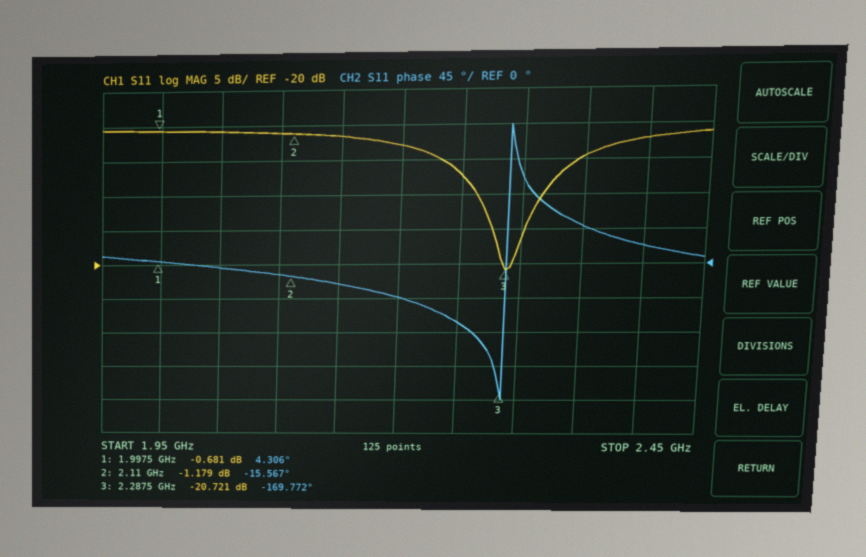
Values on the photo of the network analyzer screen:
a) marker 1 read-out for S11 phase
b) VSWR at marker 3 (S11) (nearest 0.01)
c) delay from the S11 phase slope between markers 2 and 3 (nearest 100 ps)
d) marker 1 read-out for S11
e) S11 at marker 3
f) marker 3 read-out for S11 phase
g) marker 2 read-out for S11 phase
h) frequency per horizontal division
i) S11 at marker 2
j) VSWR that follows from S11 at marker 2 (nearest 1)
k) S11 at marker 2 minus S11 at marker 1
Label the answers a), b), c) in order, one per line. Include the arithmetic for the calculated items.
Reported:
a) 4.306°
b) (1 + 0.0920)/(1 − 0.0920) ≈ 1.20
c) −(-169.772° − (-15.567°))/(360° × 177.5 MHz) ≈ 2.4 ns
d) -0.681 dB
e) -20.721 dB
f) -169.772°
g) -15.567°
h) 50 MHz
i) -1.179 dB
j) (1 + 0.8731)/(1 − 0.8731) ≈ 15
k) -1.179 − (-0.681) = -0.498 dB
